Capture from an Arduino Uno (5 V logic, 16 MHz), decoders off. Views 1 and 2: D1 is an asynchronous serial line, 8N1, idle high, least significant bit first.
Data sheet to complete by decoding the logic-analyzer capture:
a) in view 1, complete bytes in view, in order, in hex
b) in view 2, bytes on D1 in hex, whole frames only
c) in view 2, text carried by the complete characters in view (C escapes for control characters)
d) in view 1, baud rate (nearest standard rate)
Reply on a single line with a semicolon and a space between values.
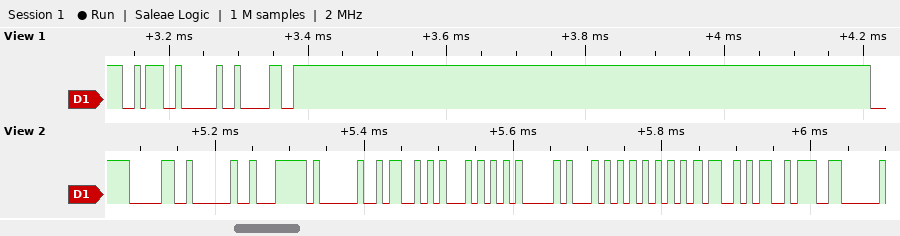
3A 20 30; 30 20 7C 20 53 54 41 54 55 53 3A; "0 | STATUS:"; 115200 baud
